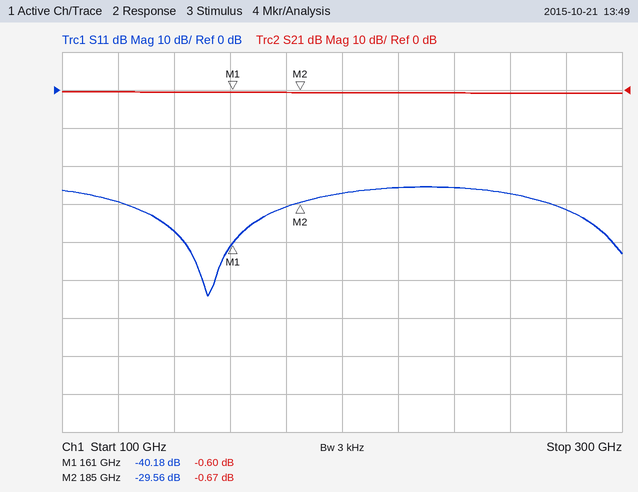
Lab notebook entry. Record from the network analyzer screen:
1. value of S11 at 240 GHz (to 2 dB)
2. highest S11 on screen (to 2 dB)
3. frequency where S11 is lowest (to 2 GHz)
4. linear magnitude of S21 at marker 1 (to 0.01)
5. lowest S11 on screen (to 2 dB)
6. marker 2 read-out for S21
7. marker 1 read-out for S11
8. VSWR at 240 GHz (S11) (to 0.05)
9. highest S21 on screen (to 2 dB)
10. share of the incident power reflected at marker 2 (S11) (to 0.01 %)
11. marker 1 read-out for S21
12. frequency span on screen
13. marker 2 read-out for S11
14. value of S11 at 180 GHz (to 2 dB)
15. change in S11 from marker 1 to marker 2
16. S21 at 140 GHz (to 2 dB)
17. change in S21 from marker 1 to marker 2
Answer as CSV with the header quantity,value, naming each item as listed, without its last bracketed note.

quantity,value
value of S11 at 240 GHz,-26 dB
highest S11 on screen,-26 dB
frequency where S11 is lowest,152 GHz
linear magnitude of S21 at marker 1,0.93
lowest S11 on screen,-54 dB
marker 2 read-out for S21,-0.67 dB
marker 1 read-out for S11,-40.18 dB
VSWR at 240 GHz (S11),1.10
highest S21 on screen,0 dB
share of the incident power reflected at marker 2 (S11),0.11 %
marker 1 read-out for S21,-0.60 dB
frequency span on screen,200 GHz
marker 2 read-out for S11,-29.56 dB
value of S11 at 180 GHz,-30 dB
change in S11 from marker 1 to marker 2,10.62 dB
S21 at 140 GHz,0 dB
change in S21 from marker 1 to marker 2,-0.07 dB
